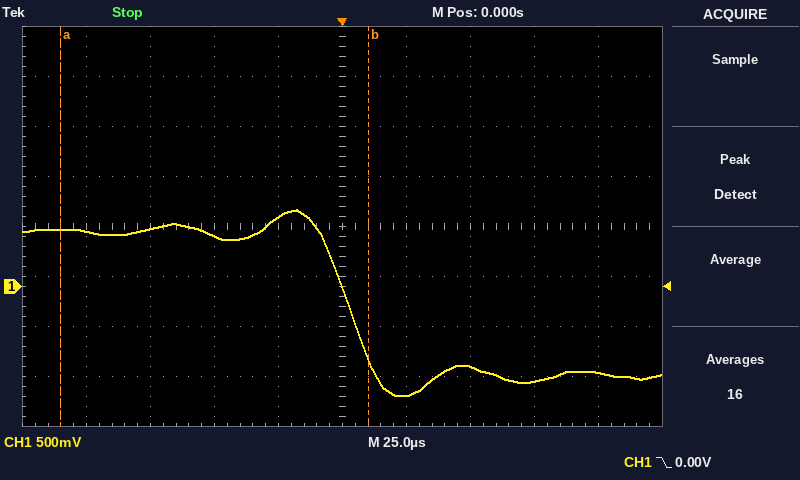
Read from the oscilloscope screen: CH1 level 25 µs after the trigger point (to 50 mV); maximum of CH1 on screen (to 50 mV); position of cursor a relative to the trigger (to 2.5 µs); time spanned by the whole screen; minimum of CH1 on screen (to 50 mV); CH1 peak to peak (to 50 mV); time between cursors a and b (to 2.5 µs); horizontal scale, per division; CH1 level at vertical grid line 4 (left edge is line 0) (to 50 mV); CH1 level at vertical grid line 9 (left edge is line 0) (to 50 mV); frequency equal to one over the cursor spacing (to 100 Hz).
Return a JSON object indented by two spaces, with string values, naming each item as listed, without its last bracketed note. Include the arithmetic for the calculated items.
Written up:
{
  "CH1 level 25 µs after the trigger point": "-1.10 V",
  "maximum of CH1 on screen": "750 mV",
  "position of cursor a relative to the trigger": "-110.0 µs",
  "time spanned by the whole screen": "250 µs",
  "minimum of CH1 on screen": "-1.10 V",
  "CH1 peak to peak": "750 mV − (-1.10 V) = 1.85 V",
  "time between cursors a and b": "120.0 µs",
  "horizontal scale, per division": "25 µs",
  "CH1 level at vertical grid line 4 (left edge is line 0)": "700 mV",
  "CH1 level at vertical grid line 9 (left edge is line 0)": "-850 mV",
  "frequency equal to one over the cursor spacing": "1 / 120.0 µs ≈ 8.3 kHz"
}
